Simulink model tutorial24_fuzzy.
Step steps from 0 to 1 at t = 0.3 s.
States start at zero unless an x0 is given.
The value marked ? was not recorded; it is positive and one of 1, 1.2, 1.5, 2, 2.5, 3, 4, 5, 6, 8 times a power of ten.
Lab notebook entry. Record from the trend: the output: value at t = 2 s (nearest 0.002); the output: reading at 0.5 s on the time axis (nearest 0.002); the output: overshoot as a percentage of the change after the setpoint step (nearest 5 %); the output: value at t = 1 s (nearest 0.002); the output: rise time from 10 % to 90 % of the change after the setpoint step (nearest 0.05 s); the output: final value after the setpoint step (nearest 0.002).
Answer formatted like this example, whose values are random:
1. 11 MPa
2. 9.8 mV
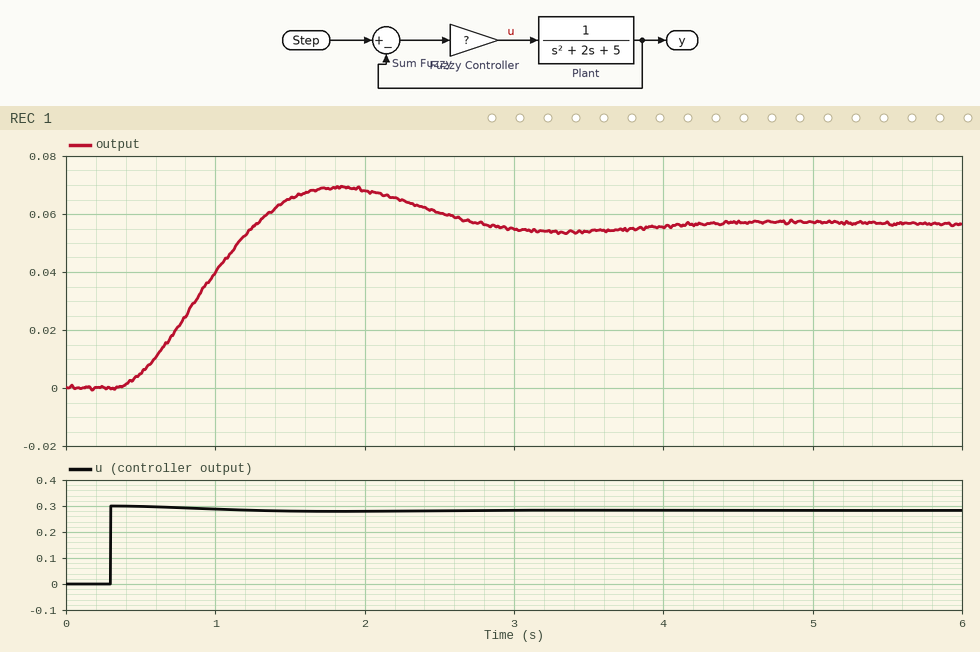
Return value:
1. 0.068
2. 0.006
3. 20 %
4. 0.040
5. 0.65 s
6. 0.056
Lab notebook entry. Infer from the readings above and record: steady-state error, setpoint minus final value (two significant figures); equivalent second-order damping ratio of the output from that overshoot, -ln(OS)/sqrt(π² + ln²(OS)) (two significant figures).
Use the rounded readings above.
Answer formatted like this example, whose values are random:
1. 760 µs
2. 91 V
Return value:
1. 0.94
2. 0.46
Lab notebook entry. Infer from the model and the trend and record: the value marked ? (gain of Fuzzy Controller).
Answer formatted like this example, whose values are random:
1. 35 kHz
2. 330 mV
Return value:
1. 0.3
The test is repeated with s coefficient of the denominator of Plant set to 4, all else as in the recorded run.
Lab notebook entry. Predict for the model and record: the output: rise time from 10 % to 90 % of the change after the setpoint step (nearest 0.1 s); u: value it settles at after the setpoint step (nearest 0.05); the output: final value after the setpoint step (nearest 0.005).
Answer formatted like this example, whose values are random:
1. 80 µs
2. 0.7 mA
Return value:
1. 1.2 s
2. 0.30
3. 0.055
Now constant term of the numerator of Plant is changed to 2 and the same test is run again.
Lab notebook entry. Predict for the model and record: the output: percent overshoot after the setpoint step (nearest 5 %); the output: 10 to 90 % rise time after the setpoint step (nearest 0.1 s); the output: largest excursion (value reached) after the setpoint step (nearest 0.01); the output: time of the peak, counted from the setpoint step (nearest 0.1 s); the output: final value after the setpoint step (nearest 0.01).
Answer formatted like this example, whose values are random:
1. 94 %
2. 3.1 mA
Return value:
1. 25 %
2. 0.6 s
3. 0.13
4. 1.5 s
5. 0.11
